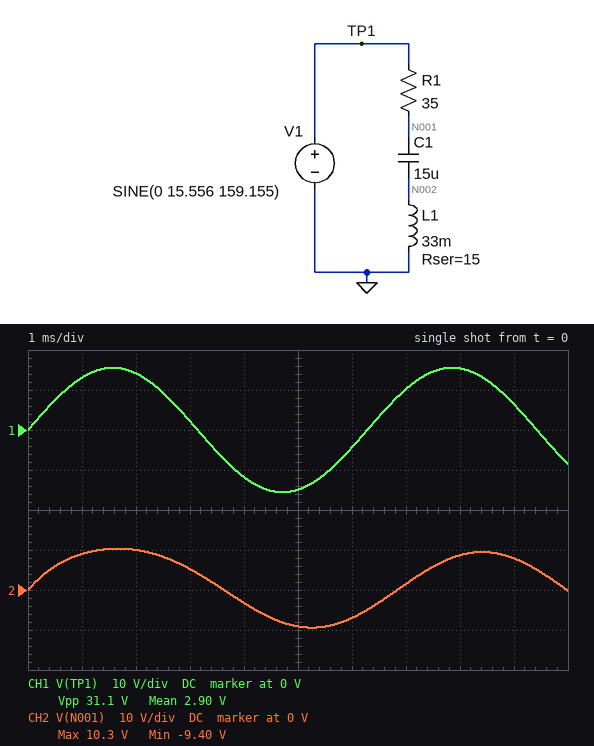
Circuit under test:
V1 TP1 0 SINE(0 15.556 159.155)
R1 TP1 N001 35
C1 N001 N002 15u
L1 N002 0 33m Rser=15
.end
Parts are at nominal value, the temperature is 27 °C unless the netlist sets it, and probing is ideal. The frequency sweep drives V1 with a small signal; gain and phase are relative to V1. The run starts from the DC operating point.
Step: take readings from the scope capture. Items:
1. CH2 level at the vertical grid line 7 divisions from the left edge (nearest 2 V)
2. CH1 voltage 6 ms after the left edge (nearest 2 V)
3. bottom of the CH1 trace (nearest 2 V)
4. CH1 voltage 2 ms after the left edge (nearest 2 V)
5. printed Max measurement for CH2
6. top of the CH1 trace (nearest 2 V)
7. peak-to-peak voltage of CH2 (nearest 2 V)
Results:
2 V
-4 V
-16 V
14 V
10.3 V
16 V
20 V
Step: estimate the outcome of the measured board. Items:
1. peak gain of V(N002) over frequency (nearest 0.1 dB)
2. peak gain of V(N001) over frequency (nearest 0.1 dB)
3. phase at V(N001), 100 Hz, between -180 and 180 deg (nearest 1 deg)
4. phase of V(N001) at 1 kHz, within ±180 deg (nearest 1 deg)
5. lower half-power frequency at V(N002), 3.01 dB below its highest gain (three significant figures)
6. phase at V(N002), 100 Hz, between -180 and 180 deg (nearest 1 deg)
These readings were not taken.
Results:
1.1 dB
0 dB
-20 deg
10 deg
190 Hz
114 deg
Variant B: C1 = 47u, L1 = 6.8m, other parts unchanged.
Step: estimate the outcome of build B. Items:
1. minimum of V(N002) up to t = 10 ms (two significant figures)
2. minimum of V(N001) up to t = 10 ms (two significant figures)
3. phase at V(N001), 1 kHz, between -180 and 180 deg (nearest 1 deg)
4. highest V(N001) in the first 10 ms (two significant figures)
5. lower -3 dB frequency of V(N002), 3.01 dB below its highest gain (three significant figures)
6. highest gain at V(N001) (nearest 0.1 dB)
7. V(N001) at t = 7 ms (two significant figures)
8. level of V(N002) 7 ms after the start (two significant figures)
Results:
-5.2 V
-5.8 V
31 deg
8.1 V
985 Hz
0 dB
1.6 V
4.8 V
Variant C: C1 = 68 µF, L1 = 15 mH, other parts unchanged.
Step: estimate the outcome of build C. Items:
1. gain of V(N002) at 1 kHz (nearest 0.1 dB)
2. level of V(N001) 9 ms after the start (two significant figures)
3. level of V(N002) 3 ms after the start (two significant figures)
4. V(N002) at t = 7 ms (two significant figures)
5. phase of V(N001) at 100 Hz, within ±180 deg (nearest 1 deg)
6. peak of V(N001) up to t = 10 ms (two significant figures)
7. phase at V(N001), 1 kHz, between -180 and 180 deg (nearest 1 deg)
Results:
-0.8 dB
2.1 V
-4.4 V
6.5 V
-27 deg
7.1 V
19 deg
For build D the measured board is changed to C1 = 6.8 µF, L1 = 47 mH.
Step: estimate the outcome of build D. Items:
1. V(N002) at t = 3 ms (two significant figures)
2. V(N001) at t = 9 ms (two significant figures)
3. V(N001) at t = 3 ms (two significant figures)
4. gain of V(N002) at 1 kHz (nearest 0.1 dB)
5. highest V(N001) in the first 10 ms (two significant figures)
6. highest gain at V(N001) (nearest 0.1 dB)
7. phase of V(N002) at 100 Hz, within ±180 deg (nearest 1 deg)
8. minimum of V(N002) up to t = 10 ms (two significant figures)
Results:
-7.8 V
9.5 V
6.0 V
0.6 dB
14 V
0 dB
139 deg
-8.8 V
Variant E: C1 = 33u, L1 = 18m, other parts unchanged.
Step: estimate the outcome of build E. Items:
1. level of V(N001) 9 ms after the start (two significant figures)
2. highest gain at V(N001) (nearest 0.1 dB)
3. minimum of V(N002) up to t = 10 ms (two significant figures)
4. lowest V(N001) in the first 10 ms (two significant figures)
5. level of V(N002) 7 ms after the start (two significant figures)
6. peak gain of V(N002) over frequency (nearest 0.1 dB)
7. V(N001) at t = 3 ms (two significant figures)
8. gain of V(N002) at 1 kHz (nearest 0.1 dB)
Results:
4.5 V
0 dB
-7.1 V
-5.7 V
6.8 V
0 dB
4.2 V
-0.4 dB
